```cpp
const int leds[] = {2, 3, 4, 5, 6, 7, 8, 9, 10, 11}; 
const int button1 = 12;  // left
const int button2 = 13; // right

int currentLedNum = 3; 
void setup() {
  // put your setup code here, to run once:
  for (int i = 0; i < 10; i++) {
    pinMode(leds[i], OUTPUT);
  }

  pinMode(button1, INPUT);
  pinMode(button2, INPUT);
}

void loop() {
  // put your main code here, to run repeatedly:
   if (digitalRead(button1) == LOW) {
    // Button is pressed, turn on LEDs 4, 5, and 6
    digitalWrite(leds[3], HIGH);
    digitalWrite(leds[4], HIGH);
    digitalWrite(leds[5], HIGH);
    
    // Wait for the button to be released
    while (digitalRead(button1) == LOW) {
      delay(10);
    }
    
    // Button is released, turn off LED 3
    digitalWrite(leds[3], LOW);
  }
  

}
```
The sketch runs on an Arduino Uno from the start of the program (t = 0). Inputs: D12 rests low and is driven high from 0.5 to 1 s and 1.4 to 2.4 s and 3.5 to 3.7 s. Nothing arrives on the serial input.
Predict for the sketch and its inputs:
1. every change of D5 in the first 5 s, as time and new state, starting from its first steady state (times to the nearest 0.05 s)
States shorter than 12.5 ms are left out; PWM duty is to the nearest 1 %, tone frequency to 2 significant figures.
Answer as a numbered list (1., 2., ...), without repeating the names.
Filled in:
1. 0 s high; 0.5 s low; 1 s high; 1.4 s low; 2.4 s high; 3.5 s low; 3.7 s high
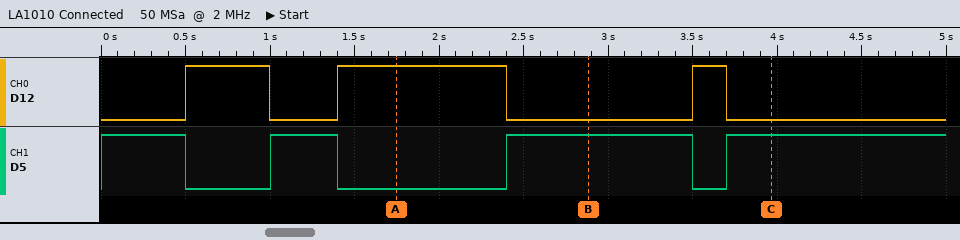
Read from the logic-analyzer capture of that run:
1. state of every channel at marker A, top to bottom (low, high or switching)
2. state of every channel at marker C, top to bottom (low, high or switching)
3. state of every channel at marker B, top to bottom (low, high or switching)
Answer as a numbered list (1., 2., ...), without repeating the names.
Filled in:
1. D12 high, D5 low
2. D12 low, D5 high
3. D12 low, D5 high
